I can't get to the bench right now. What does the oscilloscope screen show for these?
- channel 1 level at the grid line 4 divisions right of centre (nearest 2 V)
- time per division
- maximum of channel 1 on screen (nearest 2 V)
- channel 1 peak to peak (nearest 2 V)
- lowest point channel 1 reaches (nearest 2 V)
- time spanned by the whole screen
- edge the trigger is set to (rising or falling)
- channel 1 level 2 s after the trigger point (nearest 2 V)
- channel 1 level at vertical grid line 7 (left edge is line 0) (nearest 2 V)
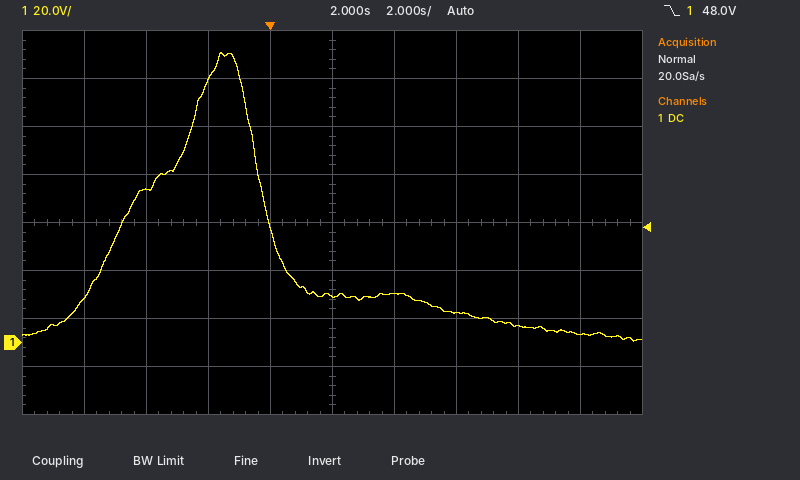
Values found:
4 V
2 s
120 V
120 V
0 V
20 s
falling
20 V
12 V
